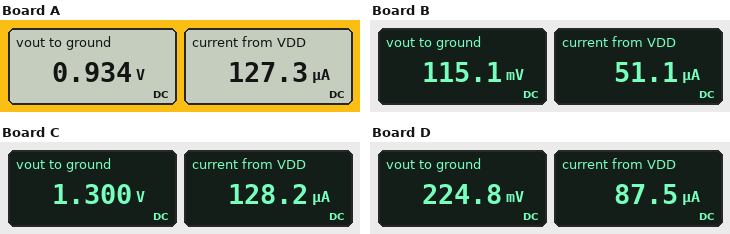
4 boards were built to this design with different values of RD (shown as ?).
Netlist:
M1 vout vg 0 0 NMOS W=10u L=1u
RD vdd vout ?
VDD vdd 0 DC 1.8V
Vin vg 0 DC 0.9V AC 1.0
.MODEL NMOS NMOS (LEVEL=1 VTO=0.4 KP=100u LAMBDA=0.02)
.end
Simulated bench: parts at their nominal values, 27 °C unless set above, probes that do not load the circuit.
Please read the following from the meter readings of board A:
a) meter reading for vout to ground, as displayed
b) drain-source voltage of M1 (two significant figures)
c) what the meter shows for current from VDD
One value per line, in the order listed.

0.934 V
930 mV
127.3 µA
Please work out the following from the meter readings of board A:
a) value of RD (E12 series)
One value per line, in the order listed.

6.8 kΩ
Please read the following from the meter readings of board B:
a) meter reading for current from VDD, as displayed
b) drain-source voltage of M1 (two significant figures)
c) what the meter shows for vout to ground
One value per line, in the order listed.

51.1 µA
120 mV
115.1 mV
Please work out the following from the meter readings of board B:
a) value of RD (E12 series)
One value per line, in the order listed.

33 kΩ
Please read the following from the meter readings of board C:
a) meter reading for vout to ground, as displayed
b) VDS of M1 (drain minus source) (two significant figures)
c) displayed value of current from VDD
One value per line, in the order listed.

1.300 V
1.3 V
128.2 µA
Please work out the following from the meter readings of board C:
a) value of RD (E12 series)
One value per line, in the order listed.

3.9 kΩ
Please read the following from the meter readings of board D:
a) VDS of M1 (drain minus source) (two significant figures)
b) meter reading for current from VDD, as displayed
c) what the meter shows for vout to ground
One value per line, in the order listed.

220 mV
87.5 µA
224.8 mV
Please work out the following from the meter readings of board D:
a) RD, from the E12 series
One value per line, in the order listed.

18 kΩ
